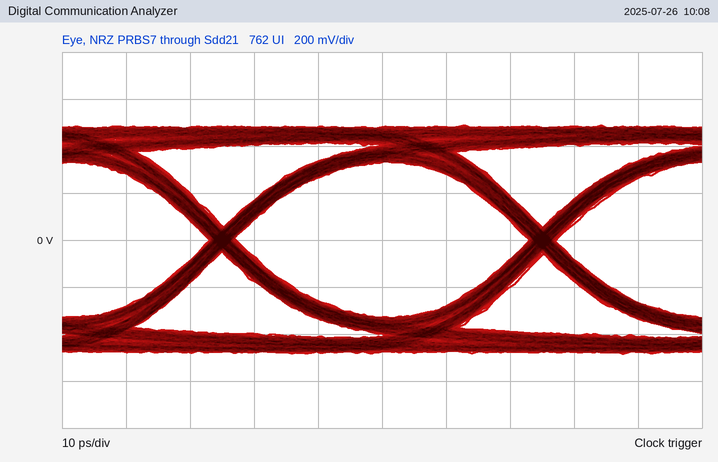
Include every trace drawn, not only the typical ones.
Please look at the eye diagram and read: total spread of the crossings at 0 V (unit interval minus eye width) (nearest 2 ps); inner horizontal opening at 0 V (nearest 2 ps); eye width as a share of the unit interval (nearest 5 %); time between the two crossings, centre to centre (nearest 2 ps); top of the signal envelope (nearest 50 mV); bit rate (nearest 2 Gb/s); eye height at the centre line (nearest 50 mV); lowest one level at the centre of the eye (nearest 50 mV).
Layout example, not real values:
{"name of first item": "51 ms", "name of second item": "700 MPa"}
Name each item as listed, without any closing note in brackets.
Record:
{"total spread of the crossings at 0 V (unit interval minus eye width)": "4 ps", "inner horizontal opening at 0 V": "46 ps", "eye width as a share of the unit interval": "90 %", "time between the two crossings, centre to centre": "50 ps", "top of the signal envelope": "500 mV", "bit rate": "20 Gb/s", "eye height at the centre line": "650 mV", "lowest one level at the centre of the eye": "350 mV"}
